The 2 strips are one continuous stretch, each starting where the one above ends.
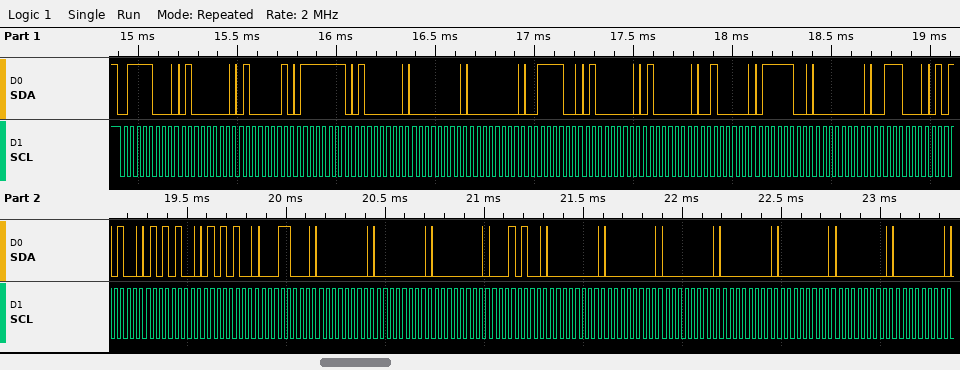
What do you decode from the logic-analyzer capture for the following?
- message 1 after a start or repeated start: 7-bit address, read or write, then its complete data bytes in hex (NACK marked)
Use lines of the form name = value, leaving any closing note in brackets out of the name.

message 1 after a start or repeated start: 7-bit address, read or write, then its complete data bytes in hex = 0x3C write: 40 41 7F 40 00 00 3C 40 40 20 7C 00 38 54 54 54 18 00 00 00 14 00 00 00 00 00 00 00
